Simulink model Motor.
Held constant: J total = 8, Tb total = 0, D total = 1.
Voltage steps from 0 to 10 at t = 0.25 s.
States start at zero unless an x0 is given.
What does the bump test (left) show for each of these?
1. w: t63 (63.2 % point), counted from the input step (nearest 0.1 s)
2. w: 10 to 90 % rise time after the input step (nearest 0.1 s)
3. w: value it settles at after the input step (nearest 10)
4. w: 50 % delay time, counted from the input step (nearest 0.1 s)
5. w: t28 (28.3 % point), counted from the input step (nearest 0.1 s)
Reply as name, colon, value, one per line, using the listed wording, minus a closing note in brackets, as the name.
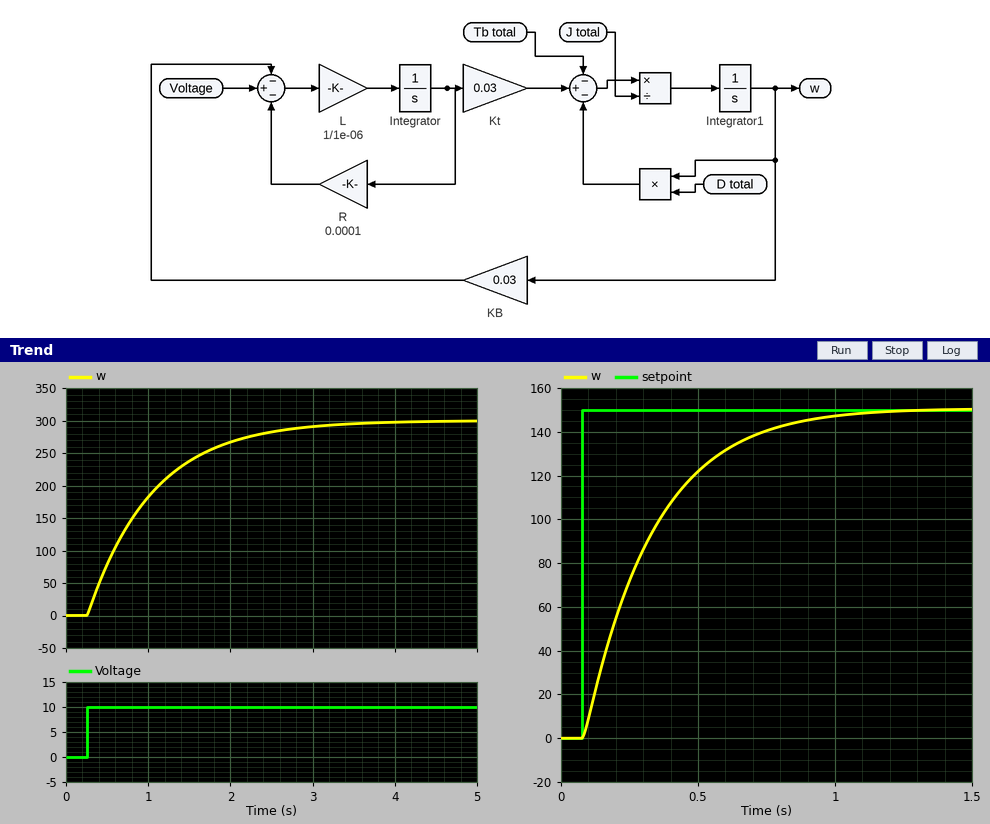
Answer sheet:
w: t63 (63.2 % point), counted from the input step: 0.8 s
w: 10 to 90 % rise time after the input step: 1.7 s
w: value it settles at after the input step: 300
w: 50 % delay time, counted from the input step: 0.6 s
w: t28 (28.3 % point), counted from the input step: 0.3 s
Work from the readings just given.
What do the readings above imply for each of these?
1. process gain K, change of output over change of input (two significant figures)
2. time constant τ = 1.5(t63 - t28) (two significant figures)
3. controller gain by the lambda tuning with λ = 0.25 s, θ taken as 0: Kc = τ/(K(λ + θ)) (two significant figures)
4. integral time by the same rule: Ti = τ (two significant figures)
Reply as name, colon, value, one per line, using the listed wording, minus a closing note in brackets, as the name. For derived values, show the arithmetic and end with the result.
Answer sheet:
process gain K, change of output over change of input: (300 - 0) / 10 = 30
time constant τ = 1.5(t63 - t28): 1.5 × (0.8 - 0.3) = 0.75 s
controller gain by the lambda tuning with λ = 0.25 s, θ taken as 0: Kc = τ/(K(λ + θ)): 0.75 / (30 × (0.25 + 0)) = 0.10
integral time by the same rule: Ti = τ: 0.75 s
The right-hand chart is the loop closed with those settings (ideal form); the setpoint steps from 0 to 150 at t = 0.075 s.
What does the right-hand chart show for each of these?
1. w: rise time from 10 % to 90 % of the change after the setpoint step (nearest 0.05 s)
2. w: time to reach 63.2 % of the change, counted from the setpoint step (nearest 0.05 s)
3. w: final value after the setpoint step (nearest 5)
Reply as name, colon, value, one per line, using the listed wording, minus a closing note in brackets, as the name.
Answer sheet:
w: rise time from 10 % to 90 % of the change after the setpoint step: 0.55 s
w: time to reach 63.2 % of the change, counted from the setpoint step: 0.25 s
w: final value after the setpoint step: 150
